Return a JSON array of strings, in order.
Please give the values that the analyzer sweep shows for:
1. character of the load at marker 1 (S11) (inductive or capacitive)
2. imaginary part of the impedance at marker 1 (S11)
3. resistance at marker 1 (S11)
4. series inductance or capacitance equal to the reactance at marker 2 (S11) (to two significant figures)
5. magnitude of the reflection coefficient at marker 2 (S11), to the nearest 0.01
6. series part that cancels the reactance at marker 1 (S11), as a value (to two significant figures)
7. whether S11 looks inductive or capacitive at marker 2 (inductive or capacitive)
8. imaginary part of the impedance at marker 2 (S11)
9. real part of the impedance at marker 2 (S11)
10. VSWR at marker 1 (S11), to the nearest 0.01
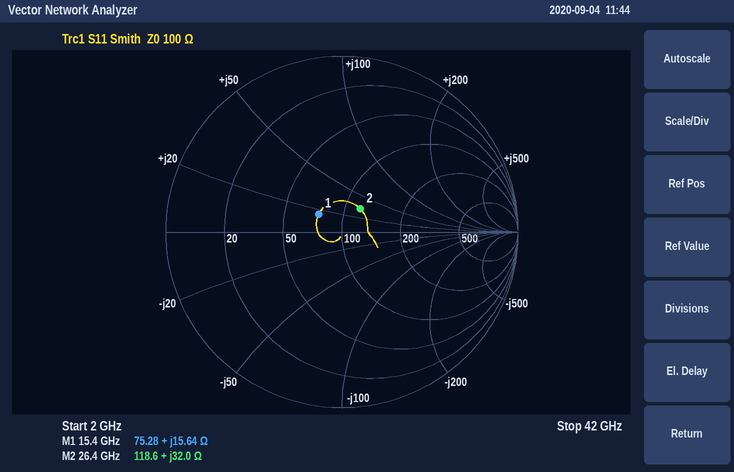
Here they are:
["inductive", "+15.64 Ω", "75.28 Ω", "190 pH", "0.17", "660 fF", "inductive", "+32.0 Ω", "118.6 Ω", "1.40"]
